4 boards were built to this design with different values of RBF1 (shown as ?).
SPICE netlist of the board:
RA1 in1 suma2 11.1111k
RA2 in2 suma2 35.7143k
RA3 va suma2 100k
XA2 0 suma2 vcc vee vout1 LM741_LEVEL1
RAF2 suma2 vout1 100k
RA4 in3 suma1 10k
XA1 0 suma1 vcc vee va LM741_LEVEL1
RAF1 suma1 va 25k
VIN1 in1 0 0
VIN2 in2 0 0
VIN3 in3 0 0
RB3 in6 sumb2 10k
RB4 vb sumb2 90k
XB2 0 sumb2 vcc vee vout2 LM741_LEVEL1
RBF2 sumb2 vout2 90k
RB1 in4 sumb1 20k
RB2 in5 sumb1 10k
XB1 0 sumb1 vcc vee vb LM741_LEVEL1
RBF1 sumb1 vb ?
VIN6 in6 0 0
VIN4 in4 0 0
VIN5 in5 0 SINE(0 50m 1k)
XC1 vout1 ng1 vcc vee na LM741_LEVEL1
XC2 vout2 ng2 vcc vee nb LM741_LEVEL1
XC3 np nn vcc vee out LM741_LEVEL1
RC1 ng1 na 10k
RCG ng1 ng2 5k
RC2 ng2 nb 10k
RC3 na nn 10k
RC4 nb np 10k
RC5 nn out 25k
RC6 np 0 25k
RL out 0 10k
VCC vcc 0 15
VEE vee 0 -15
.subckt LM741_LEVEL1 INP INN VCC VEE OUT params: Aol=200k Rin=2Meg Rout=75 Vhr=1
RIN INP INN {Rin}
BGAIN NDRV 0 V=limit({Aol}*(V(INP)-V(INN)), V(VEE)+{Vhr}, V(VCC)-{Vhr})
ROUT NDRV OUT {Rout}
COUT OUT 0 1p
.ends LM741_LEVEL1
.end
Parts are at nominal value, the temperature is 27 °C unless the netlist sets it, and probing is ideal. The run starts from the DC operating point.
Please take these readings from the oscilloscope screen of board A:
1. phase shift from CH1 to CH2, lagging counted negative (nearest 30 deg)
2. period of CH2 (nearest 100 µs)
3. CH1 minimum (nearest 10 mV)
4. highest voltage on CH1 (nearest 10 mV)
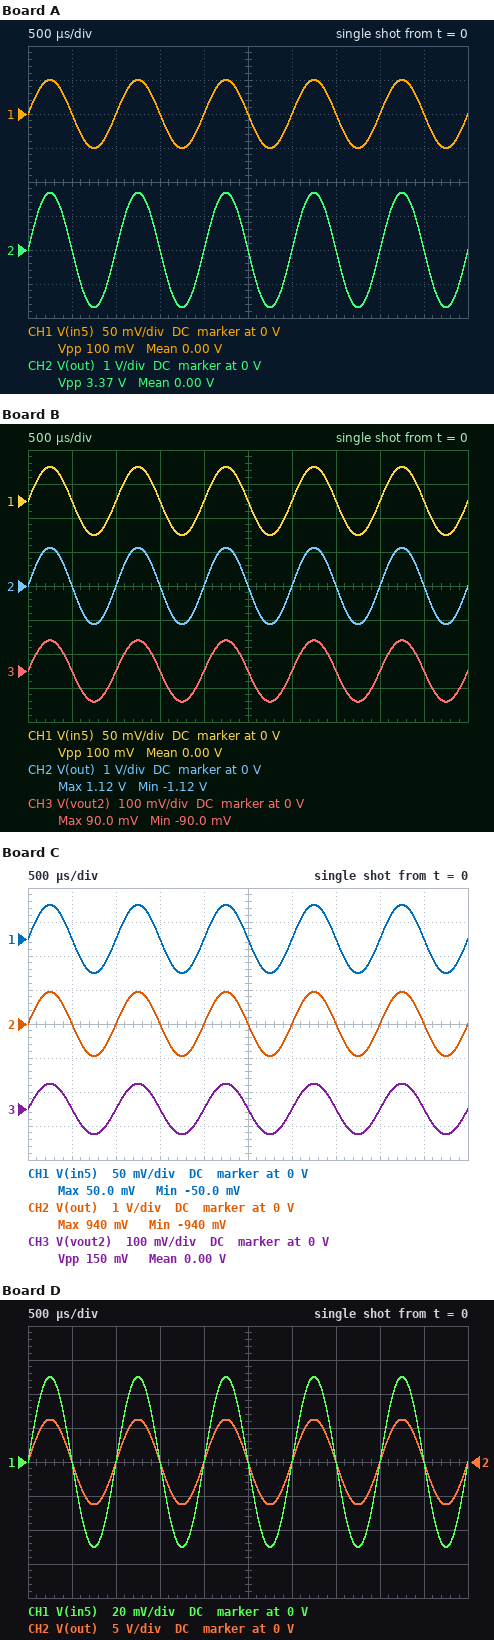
0 deg
1.0 ms
-50 mV
50 mV
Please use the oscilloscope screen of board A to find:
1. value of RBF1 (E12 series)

27 kΩ
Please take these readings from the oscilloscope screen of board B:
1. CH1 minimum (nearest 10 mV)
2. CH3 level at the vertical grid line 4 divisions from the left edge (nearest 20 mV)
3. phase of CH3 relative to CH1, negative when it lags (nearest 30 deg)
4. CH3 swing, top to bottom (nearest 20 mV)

-50 mV
0 V
0 deg
180 mV
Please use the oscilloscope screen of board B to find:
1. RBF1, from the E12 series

18 kΩ
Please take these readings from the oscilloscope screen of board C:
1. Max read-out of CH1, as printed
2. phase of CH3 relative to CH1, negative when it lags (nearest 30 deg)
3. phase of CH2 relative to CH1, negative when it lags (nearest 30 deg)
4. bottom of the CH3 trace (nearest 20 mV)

50.0 mV
0 deg
0 deg
-80 mV
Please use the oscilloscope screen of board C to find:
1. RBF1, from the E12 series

15 kΩ
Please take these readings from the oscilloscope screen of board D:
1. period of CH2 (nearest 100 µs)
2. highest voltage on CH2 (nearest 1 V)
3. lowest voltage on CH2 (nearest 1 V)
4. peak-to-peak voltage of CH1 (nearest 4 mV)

1.0 ms
6 V
-6 V
100 mV
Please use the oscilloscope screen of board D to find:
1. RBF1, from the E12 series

100 kΩ
